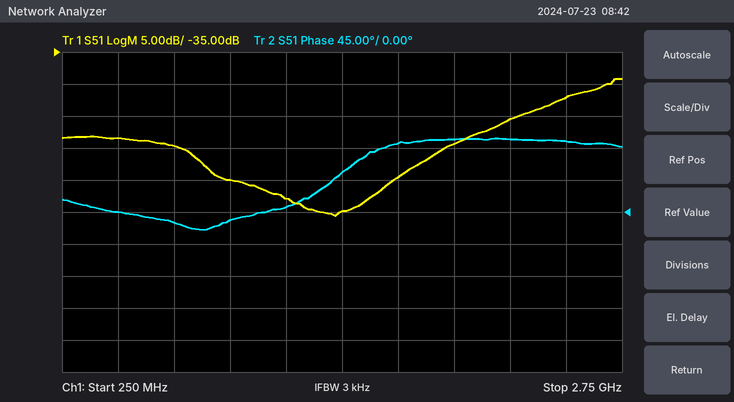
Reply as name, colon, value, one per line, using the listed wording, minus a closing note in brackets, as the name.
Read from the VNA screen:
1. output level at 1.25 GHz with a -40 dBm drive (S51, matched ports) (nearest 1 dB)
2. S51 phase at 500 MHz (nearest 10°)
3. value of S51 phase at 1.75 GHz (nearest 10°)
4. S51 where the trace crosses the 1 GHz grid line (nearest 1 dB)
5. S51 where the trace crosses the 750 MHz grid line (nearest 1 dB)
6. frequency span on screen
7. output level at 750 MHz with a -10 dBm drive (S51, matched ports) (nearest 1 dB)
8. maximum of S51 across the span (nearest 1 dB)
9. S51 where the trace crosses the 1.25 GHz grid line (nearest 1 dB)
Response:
output level at 1.25 GHz with a -40 dBm drive (S51, matched ports): -98 dBm
S51 phase at 500 MHz: 0°
value of S51 phase at 1.75 GHz: 100°
S51 where the trace crosses the 1 GHz grid line: -55 dB
S51 where the trace crosses the 750 MHz grid line: -50 dB
frequency span on screen: 2.5 GHz
output level at 750 MHz with a -10 dBm drive (S51, matched ports): -60 dBm
maximum of S51 across the span: -39 dB
S51 where the trace crosses the 1.25 GHz grid line: -58 dB
